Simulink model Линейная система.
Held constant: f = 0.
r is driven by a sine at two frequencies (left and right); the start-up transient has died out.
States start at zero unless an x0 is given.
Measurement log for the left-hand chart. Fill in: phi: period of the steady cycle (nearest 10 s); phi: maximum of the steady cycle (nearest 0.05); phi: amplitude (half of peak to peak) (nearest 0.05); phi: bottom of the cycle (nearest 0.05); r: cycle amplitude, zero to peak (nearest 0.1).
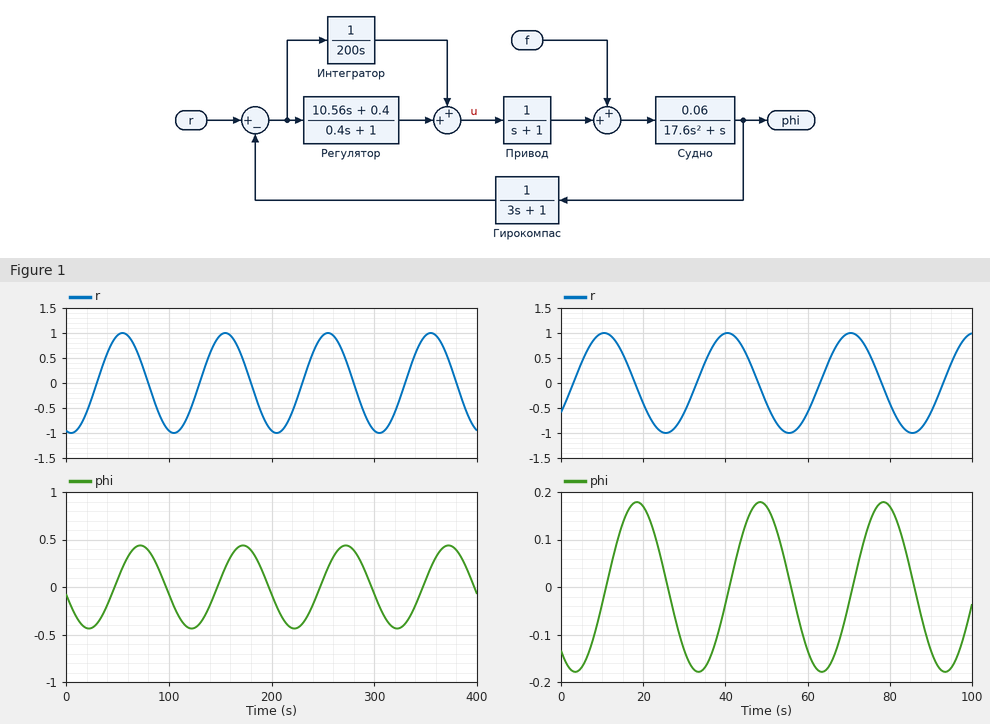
100 s
0.45
0.45
-0.45
1.0
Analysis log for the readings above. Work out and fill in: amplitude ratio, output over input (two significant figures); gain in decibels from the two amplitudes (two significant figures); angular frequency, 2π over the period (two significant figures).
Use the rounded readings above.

0.45
-6.9 dB
0.063 rad/s
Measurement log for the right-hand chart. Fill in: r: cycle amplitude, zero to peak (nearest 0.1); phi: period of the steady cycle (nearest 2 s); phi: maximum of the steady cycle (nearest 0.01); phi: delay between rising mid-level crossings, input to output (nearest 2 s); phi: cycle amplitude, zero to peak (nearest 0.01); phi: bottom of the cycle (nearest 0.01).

1.0
30 s
0.18
8 s
0.18
-0.18
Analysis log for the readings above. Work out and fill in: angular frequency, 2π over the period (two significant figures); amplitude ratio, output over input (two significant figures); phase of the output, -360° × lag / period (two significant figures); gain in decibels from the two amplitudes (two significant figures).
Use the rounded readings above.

0.21 rad/s
0.18
-96°
-15 dB
